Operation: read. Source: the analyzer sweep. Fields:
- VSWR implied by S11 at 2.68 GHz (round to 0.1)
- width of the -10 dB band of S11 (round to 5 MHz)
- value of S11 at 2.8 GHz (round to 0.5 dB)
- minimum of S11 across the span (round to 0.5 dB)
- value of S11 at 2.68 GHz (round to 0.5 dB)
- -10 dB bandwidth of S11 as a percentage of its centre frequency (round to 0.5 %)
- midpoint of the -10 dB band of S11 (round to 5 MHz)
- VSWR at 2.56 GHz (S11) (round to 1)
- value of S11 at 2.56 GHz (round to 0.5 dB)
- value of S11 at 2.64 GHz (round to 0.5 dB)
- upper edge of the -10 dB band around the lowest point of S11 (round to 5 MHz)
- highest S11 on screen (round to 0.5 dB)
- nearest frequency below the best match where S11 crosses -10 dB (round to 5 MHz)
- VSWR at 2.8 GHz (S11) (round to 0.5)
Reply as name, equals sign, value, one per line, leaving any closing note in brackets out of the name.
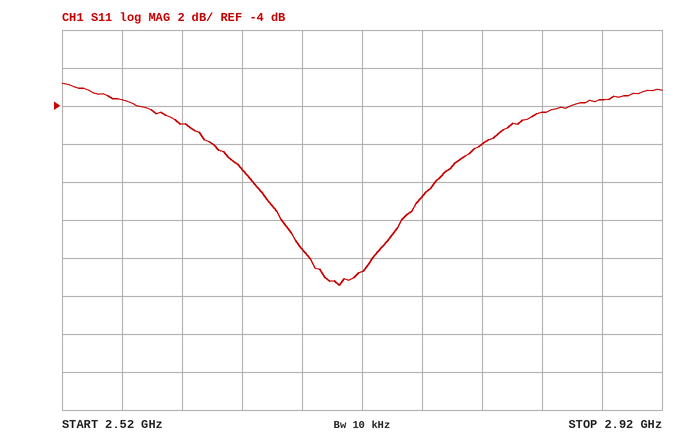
VSWR implied by S11 at 2.68 GHz = 1.7
width of the -10 dB band of S11 = 80 MHz
value of S11 at 2.8 GHz = -6.0 dB
minimum of S11 across the span = -13.5 dB
value of S11 at 2.68 GHz = -11.5 dB
-10 dB bandwidth of S11 as a percentage of its centre frequency = 3.0 %
midpoint of the -10 dB band of S11 = 2.705 GHz
VSWR at 2.56 GHz (S11) = 5
value of S11 at 2.56 GHz = -3.5 dB
value of S11 at 2.64 GHz = -7.5 dB
upper edge of the -10 dB band around the lowest point of S11 = 2.745 GHz
highest S11 on screen = -3.0 dB
nearest frequency below the best match where S11 crosses -10 dB = 2.665 GHz
VSWR at 2.8 GHz (S11) = 3.0
